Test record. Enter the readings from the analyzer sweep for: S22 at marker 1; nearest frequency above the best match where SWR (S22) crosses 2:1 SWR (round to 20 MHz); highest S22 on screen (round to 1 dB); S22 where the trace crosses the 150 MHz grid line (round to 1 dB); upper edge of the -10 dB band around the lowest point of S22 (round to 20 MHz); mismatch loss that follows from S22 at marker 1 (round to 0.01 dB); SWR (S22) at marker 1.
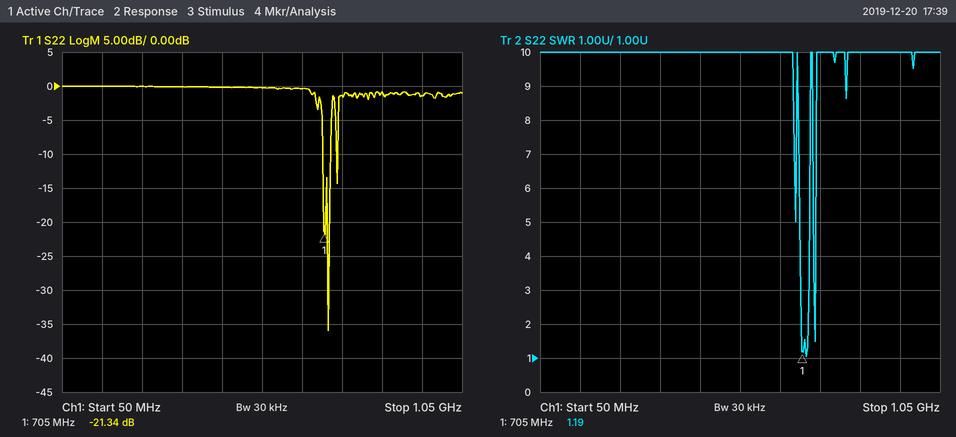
-21.34 dB
720 MHz
0 dB
0 dB
720 MHz
0.03 dB
1.19
